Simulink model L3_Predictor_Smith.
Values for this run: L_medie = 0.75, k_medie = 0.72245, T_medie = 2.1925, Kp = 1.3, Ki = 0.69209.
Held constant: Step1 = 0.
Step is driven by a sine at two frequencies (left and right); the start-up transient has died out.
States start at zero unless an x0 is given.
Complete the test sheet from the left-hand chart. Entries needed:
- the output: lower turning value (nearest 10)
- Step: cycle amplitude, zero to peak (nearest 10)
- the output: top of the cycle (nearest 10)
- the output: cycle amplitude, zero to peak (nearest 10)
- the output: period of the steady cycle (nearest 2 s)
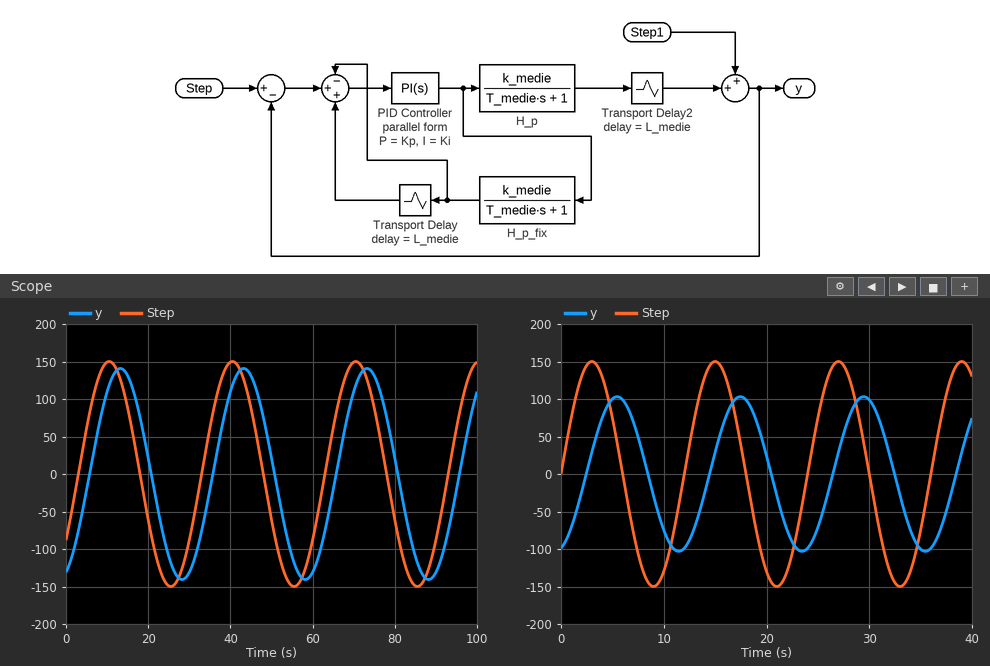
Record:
-140
150
140
140
30 s
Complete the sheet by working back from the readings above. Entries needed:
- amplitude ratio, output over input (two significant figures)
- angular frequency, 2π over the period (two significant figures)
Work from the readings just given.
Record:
0.93
0.21 rad/s
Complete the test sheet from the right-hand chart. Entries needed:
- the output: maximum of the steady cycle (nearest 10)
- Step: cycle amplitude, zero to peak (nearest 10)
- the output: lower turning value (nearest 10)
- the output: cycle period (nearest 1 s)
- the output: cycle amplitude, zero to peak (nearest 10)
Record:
100
150
-100
12 s
100
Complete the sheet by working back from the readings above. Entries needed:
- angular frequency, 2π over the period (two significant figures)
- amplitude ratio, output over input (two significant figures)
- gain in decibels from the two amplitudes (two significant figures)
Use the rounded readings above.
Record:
0.52 rad/s
0.67
-3.5 dB
